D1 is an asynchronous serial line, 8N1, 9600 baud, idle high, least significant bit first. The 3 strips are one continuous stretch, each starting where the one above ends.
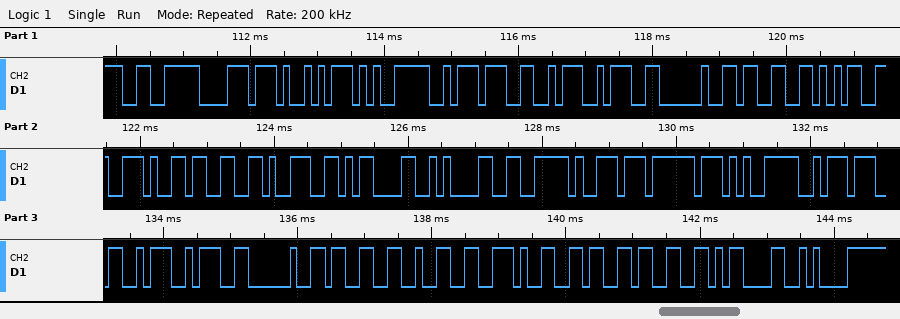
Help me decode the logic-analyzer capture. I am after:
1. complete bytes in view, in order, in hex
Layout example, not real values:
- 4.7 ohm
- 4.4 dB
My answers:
- E6 B8 A9 E5 BA A6 3A 20 33 35 2E 33 39 0D 0A E6 B9 BF E5 BA A6 3A 20 33 32 2E 36 33 0D 0A
